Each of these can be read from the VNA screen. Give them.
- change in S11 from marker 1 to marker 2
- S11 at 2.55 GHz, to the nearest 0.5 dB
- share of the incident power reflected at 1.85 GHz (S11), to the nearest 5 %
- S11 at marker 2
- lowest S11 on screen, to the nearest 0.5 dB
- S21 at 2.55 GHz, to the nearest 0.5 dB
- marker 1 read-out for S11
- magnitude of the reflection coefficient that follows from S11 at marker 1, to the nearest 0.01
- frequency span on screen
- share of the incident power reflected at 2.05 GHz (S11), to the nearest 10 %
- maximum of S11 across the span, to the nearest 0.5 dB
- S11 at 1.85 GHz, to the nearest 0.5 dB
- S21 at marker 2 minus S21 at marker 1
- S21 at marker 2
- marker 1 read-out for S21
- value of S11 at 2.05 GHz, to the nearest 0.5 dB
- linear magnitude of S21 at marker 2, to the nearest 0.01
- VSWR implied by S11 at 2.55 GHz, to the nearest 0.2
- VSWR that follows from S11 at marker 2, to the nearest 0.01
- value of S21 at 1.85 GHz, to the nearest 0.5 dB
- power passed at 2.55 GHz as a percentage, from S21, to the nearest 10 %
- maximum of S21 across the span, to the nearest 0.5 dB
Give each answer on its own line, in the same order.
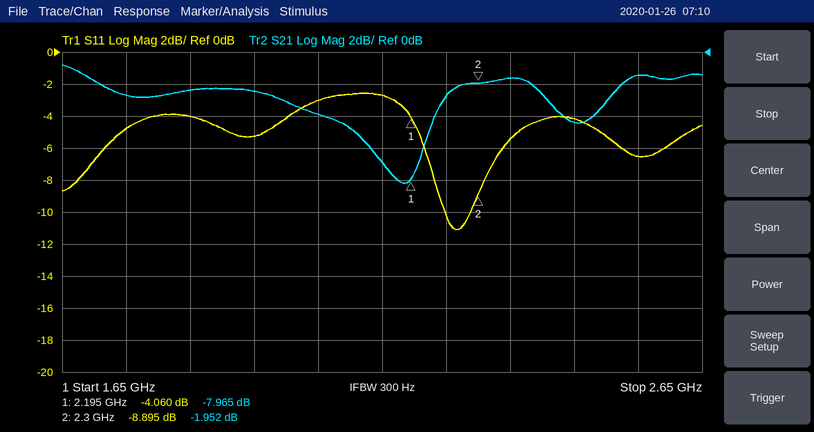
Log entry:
-4.835 dB
-6.5 dB
40 %
-8.895 dB
-11.0 dB
-1.5 dB
-4.060 dB
0.63
1 GHz
50 %
-2.5 dB
-4.0 dB
6.013 dB
-1.952 dB
-7.965 dB
-3.0 dB
0.80
2.8
2.12
-2.5 dB
70 %
-1.0 dB
